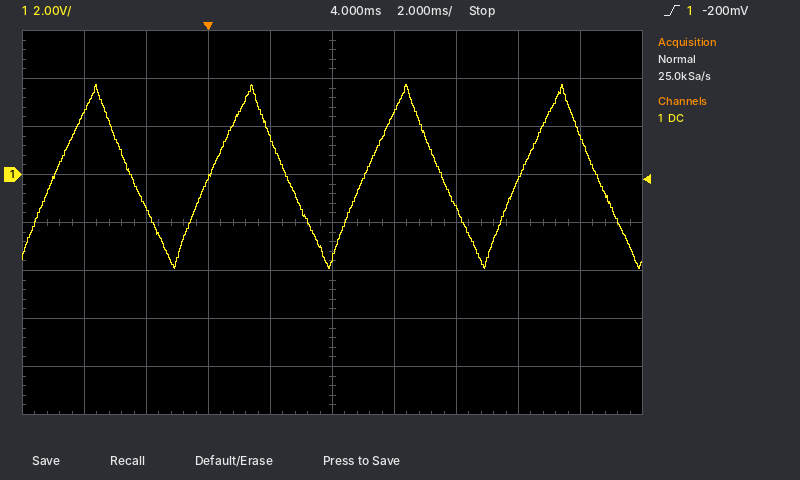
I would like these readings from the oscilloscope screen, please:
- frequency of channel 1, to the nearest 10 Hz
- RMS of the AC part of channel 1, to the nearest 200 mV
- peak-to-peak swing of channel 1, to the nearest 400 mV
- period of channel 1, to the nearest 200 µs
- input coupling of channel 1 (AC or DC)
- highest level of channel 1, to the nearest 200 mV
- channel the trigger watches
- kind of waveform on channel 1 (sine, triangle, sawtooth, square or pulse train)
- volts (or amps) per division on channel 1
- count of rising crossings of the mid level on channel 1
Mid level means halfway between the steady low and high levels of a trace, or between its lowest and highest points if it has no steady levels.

200 Hz
2.2 V
7.6 V
5.0 ms
DC
3.8 V
channel 1
triangle
2 V
4
